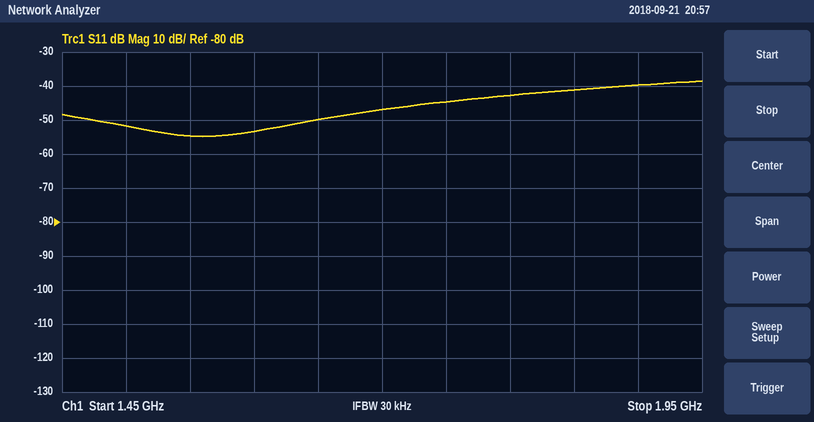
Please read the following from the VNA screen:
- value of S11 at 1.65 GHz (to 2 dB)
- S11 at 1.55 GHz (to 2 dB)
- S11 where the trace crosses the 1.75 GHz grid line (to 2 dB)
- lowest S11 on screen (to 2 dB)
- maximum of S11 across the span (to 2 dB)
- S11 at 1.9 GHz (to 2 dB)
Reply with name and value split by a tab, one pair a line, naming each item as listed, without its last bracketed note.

value of S11 at 1.65 GHz	-50 dB
S11 at 1.55 GHz	-54 dB
S11 where the trace crosses the 1.75 GHz grid line	-44 dB
lowest S11 on screen	-54 dB
maximum of S11 across the span	-38 dB
S11 at 1.9 GHz	-40 dB
